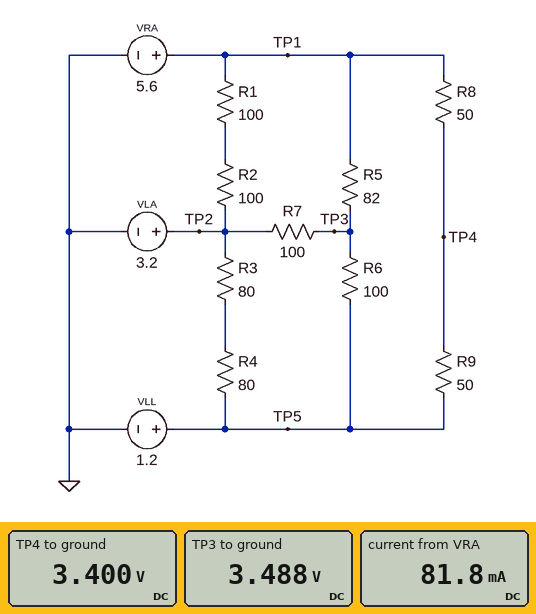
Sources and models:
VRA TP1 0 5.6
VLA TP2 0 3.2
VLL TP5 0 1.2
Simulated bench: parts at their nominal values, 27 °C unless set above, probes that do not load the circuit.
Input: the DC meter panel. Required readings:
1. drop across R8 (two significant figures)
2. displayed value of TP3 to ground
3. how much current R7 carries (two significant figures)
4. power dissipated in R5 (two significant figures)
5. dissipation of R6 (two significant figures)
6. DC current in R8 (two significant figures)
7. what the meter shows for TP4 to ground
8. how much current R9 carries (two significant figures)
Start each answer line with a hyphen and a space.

- 2.2 V
- 3.488 V
- 2.9 mA
- 54 mW
- 52 mW
- 44 mA
- 3.400 V
- 44 mA
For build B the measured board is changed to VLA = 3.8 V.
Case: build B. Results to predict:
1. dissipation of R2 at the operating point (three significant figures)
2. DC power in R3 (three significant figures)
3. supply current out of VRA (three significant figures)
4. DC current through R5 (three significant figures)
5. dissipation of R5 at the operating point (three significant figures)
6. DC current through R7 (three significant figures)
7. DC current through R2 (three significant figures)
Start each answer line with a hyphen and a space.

- 8.10 mW
- 21.1 mW
- 76.5 mA
- 23.5 mA
- 45.2 mW
- 1.26 mA
- 9.00 mA
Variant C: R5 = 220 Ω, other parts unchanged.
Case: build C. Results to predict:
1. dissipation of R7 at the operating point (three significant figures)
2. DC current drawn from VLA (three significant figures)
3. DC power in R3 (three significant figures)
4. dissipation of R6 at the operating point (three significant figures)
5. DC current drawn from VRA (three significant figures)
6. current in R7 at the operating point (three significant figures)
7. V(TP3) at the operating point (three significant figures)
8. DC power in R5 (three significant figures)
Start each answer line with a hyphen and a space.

- 1.37 mW
- 4.20 mA
- 12.5 mW
- 26.6 mW
- 68.6 mA
- 3.70 mA
- 2.83 V
- 34.9 mW
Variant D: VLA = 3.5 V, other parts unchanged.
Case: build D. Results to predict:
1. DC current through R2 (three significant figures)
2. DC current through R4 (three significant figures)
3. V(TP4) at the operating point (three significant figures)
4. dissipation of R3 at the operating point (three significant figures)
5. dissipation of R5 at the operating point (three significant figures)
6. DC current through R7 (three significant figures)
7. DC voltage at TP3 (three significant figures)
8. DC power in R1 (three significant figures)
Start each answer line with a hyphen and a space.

- 10.5 mA
- 14.4 mA
- 3.40 V
- 16.5 mW
- 49.7 mW
- 811 µA
- 3.58 V
- 11.0 mW
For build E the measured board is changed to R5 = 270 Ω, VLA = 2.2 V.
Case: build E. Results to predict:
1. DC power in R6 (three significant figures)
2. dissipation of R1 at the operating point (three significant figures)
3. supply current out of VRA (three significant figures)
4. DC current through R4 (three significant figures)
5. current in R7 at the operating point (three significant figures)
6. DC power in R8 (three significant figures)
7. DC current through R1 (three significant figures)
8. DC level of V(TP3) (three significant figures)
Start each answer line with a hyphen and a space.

- 12.3 mW
- 28.9 mW
- 73.2 mA
- 6.25 mA
- 1.09 mA
- 96.8 mW
- 17.0 mA
- 2.31 V
